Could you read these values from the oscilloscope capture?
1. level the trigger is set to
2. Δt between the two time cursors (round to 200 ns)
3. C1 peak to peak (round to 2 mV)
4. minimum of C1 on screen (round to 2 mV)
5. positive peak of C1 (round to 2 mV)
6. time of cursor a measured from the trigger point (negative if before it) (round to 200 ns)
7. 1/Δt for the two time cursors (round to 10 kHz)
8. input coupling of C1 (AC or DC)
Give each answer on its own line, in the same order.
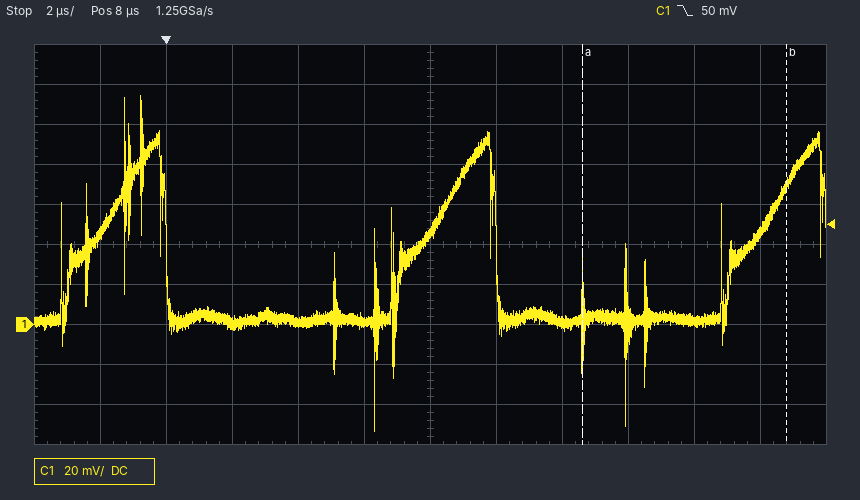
50 mV
6.2 µs
168 mV
-54 mV
114 mV
+12.6 µs
160 kHz
DC
